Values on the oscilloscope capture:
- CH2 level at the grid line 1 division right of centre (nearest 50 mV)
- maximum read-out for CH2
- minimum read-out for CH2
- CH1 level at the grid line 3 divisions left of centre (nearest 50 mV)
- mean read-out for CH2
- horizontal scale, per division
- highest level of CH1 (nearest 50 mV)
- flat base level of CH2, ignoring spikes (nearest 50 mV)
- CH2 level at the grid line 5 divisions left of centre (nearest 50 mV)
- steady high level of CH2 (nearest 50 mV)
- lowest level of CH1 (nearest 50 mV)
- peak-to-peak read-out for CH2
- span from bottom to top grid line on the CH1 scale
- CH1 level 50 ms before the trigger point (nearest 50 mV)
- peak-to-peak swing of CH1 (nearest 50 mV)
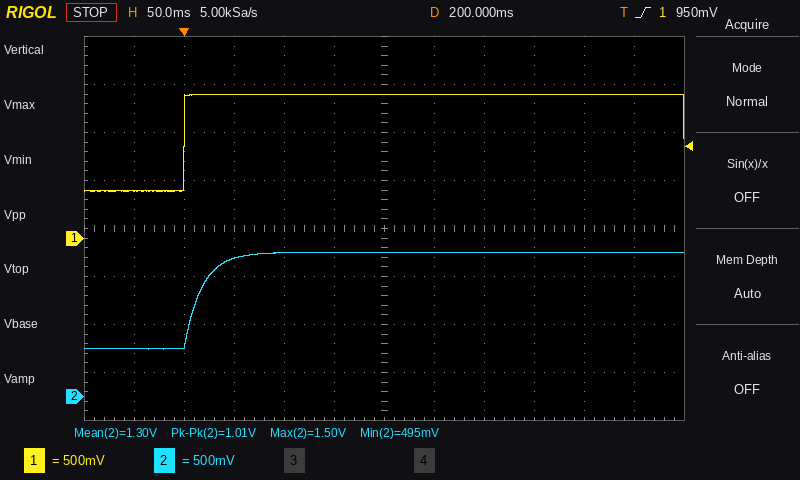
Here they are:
1.50 V
1.50 V
495 mV
1.50 V
1.30 V
50 ms
1.50 V
500 mV
500 mV
1.50 V
500 mV
1.01 V
4 V
500 mV
1.00 V
